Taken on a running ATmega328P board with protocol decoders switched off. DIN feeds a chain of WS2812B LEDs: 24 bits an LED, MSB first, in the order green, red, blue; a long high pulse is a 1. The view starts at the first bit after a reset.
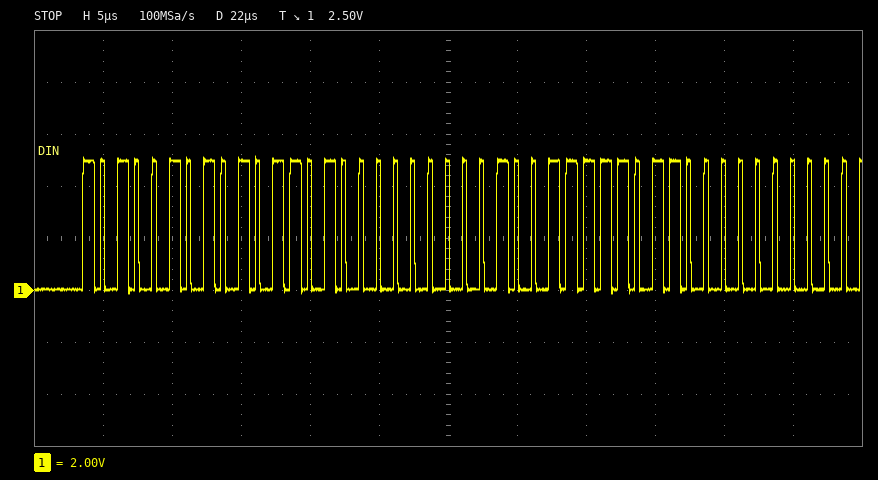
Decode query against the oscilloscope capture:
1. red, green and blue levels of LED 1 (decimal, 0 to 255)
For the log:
90, 165, 0
